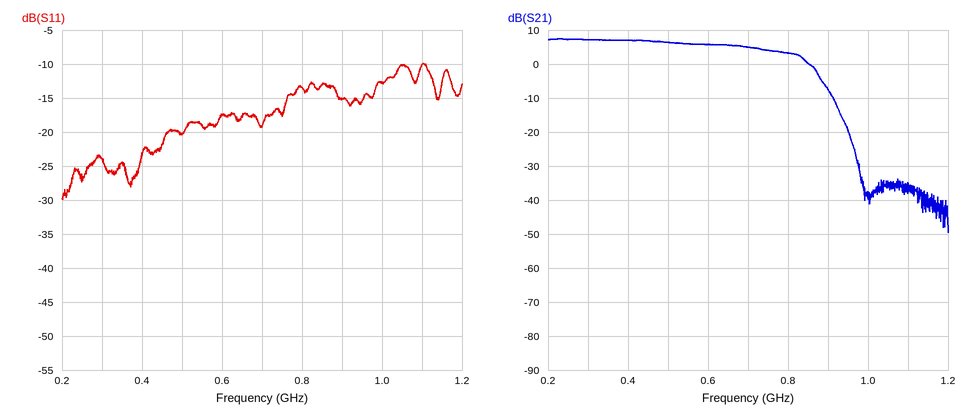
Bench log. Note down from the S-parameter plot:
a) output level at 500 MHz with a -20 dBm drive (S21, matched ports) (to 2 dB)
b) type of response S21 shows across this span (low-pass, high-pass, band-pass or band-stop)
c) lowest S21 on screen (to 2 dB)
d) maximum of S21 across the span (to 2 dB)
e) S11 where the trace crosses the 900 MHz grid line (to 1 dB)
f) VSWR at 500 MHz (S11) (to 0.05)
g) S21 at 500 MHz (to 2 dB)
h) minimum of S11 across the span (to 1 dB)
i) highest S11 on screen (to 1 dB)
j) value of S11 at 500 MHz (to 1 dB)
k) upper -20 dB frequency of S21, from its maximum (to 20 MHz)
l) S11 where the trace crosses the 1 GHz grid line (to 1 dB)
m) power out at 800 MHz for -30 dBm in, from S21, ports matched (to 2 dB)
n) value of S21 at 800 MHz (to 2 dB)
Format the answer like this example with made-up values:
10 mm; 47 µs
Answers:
-14 dBm; low-pass; -50 dB; 8 dB; -15 dB; 1.20; 6 dB; -30 dB; -10 dB; -20 dB; 920 MHz; -13 dB; -26 dBm; 4 dB
